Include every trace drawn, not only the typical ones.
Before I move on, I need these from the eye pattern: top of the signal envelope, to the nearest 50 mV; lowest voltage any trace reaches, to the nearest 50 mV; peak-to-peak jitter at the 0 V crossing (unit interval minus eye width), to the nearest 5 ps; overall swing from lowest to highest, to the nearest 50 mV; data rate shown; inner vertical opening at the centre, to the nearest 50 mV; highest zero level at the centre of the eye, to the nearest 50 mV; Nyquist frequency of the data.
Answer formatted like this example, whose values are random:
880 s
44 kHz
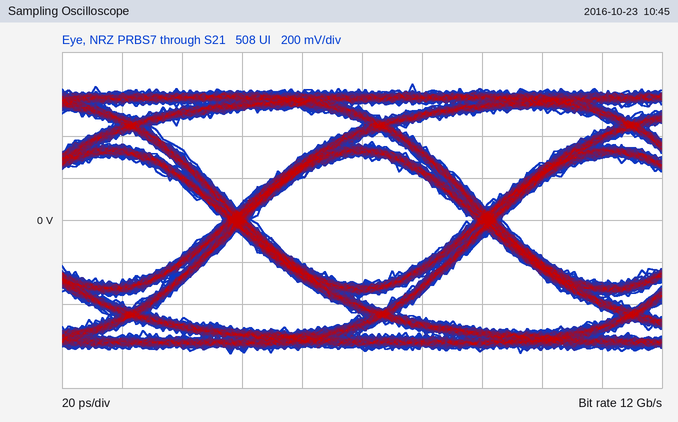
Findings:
650 mV
-650 mV
10 ps
1.30 V
12 Gb/s
600 mV
-300 mV
6 GHz
